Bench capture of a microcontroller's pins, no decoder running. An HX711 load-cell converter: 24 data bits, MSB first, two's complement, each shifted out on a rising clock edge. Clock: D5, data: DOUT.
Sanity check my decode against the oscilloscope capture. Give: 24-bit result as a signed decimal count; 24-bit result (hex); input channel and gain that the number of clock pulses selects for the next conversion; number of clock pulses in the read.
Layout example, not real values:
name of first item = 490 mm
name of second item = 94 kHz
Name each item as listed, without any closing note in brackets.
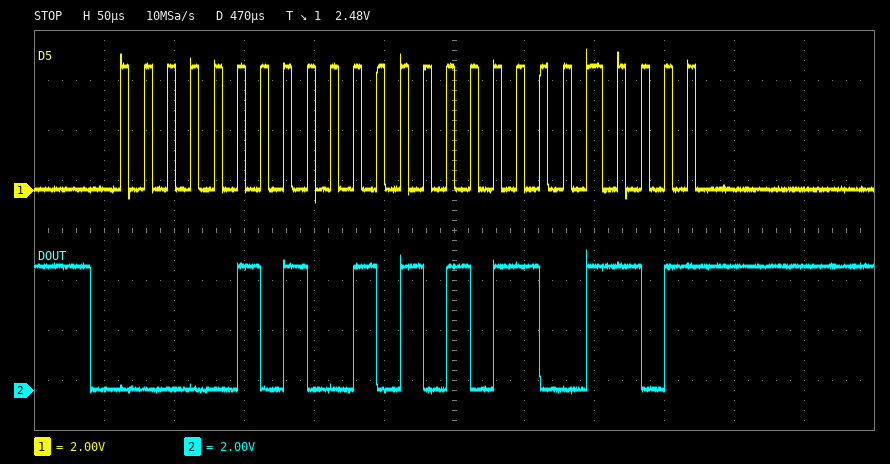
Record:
24-bit result as a signed decimal count = 338637
24-bit result = 0x052ACD
input channel and gain that the number of clock pulses selects for the next conversion = channel A, gain 128
number of clock pulses in the read = 25
